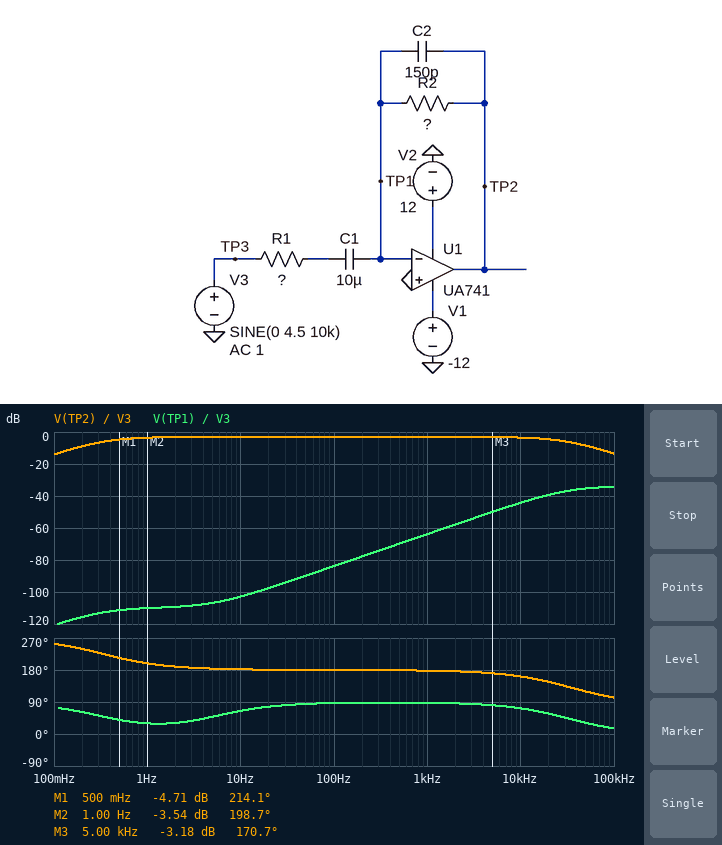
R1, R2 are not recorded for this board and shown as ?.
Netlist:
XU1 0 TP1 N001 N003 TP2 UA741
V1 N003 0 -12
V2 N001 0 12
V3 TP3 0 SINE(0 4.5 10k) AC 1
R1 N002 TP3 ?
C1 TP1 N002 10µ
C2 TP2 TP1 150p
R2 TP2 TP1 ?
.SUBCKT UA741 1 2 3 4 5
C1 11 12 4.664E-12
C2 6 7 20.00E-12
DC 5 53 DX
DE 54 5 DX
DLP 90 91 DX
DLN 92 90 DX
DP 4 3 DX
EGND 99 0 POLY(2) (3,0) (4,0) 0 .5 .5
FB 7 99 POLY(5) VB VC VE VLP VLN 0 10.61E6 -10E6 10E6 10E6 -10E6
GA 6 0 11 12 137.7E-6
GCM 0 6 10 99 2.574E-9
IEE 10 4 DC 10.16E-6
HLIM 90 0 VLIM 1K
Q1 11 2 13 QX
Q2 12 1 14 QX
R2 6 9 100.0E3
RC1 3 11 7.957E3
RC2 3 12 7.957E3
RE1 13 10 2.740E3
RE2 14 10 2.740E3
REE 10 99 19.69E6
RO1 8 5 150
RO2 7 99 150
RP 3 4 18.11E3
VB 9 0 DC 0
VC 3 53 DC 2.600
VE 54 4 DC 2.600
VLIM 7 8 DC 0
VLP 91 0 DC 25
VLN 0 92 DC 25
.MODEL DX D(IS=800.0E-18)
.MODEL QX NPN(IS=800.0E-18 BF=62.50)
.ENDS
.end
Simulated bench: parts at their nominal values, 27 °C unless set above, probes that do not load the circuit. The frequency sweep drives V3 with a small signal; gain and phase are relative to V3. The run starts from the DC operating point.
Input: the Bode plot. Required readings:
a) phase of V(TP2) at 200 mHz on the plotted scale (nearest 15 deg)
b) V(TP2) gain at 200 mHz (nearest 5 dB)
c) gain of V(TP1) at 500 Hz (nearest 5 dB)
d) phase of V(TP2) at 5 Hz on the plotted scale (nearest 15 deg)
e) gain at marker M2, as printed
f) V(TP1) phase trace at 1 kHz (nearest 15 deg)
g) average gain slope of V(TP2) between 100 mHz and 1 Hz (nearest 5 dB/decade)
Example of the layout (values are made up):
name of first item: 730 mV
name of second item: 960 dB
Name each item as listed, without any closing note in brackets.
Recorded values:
phase of V(TP2) at 200 mHz on the plotted scale: 240 deg
V(TP2) gain at 200 mHz: -10 dB
gain of V(TP1) at 500 Hz: -70 dB
phase of V(TP2) at 5 Hz on the plotted scale: 180 deg
gain at marker M2, as printed: -3.54 dB
V(TP1) phase trace at 1 kHz: 90 deg
average gain slope of V(TP2) between 100 mHz and 1 Hz: 10 dB/decade
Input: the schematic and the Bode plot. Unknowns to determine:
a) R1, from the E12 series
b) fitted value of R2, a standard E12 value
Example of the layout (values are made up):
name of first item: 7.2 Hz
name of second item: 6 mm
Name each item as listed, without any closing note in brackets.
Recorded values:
R1, from the E12 series: 47 kΩ
fitted value of R2, a standard E12 value: 33 kΩ
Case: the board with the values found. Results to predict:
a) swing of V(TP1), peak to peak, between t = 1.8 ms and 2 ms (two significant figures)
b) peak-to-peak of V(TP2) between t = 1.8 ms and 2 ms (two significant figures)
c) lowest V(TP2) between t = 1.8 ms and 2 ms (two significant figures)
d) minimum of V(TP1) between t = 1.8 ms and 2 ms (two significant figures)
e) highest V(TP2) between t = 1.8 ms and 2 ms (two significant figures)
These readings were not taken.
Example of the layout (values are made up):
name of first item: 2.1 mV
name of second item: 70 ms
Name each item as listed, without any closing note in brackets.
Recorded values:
swing of V(TP1), peak to peak, between t = 1.8 ms and 2 ms: 57 mV
peak-to-peak of V(TP2) between t = 1.8 ms and 2 ms: 6.0 V
lowest V(TP2) between t = 1.8 ms and 2 ms: -3.0 V
minimum of V(TP1) between t = 1.8 ms and 2 ms: -28 mV
highest V(TP2) between t = 1.8 ms and 2 ms: 3.0 V
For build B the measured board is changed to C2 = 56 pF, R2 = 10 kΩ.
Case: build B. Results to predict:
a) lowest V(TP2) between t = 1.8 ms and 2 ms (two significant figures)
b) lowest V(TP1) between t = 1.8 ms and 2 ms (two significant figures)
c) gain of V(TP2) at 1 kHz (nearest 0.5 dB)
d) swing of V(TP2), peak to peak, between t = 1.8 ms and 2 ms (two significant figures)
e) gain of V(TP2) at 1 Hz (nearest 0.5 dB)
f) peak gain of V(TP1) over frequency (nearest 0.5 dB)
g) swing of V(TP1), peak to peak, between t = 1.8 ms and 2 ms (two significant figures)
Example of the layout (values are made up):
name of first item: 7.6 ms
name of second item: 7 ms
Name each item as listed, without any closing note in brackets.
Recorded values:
lowest V(TP2) between t = 1.8 ms and 2 ms: -960 mV
lowest V(TP1) between t = 1.8 ms and 2 ms: -8.9 mV
gain of V(TP2) at 1 kHz: -13.5 dB
swing of V(TP2), peak to peak, between t = 1.8 ms and 2 ms: 1.9 V
gain of V(TP2) at 1 Hz: -14.0 dB
peak gain of V(TP1) over frequency: -25.5 dB
swing of V(TP1), peak to peak, between t = 1.8 ms and 2 ms: 18 mV
